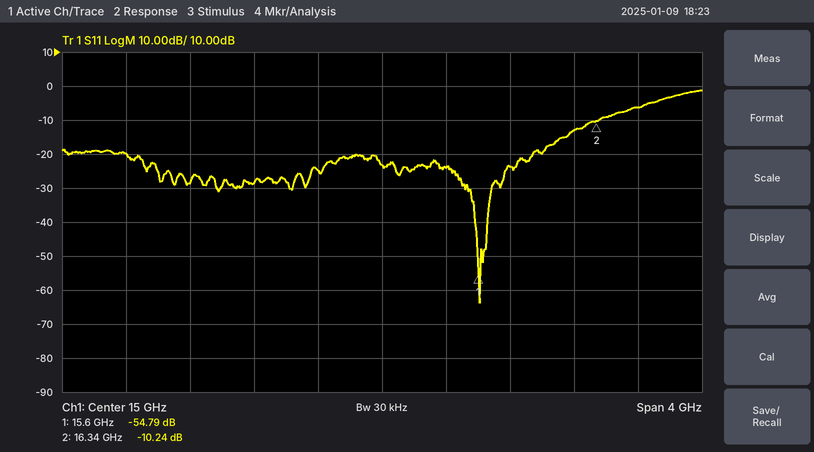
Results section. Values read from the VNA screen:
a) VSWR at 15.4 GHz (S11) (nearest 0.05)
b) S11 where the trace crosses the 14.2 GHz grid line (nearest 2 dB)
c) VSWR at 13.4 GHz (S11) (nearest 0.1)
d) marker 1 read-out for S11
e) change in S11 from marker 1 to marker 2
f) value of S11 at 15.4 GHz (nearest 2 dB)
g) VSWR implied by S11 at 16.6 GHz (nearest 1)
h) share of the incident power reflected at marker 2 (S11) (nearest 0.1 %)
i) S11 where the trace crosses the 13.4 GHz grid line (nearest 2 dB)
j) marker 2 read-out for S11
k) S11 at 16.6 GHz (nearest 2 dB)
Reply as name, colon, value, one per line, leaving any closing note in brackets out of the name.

VSWR at 15.4 GHz (S11): 1.15
S11 where the trace crosses the 14.2 GHz grid line: -28 dB
VSWR at 13.4 GHz (S11): 1.2
marker 1 read-out for S11: -54.79 dB
change in S11 from marker 1 to marker 2: 44.55 dB
value of S11 at 15.4 GHz: -24 dB
VSWR implied by S11 at 16.6 GHz: 3
share of the incident power reflected at marker 2 (S11): 9.5 %
S11 where the trace crosses the 13.4 GHz grid line: -20 dB
marker 2 read-out for S11: -10.24 dB
S11 at 16.6 GHz: -6 dB
